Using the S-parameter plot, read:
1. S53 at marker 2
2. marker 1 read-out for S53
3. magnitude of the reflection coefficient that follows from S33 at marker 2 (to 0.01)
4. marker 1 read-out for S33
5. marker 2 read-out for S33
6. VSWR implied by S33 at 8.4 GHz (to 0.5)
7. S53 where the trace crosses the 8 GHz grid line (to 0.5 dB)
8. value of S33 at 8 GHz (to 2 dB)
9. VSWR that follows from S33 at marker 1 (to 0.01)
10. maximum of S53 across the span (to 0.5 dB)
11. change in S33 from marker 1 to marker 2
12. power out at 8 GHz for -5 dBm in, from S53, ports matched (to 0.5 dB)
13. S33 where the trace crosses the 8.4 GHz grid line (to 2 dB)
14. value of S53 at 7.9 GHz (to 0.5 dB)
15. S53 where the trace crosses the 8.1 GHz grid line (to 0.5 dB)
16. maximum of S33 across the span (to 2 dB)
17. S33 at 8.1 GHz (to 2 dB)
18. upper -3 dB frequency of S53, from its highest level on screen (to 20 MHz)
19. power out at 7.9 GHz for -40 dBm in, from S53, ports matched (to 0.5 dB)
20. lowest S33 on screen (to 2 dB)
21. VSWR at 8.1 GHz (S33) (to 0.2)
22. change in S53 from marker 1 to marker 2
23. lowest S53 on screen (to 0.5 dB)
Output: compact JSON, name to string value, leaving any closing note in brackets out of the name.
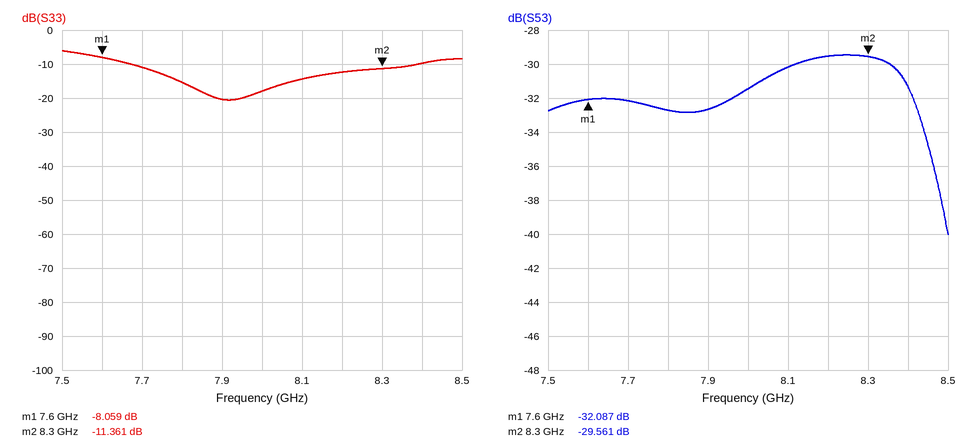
{"S53 at marker 2": "-29.561 dB", "marker 1 read-out for S53": "-32.087 dB", "magnitude of the reflection coefficient that follows from S33 at marker 2": "0.27", "marker 1 read-out for S33": "-8.059 dB", "marker 2 read-out for S33": "-11.361 dB", "VSWR implied by S33 at 8.4 GHz": "2.0", "S53 where the trace crosses the 8 GHz grid line": "-31.5 dB", "value of S33 at 8 GHz": "-18 dB", "VSWR that follows from S33 at marker 1": "2.31", "maximum of S53 across the span": "-29.5 dB", "change in S33 from marker 1 to marker 2": "-3.302 dB", "power out at 8 GHz for -5 dBm in, from S53, ports matched": "-36.5 dBm", "S33 where the trace crosses the 8.4 GHz grid line": "-10 dB", "value of S53 at 7.9 GHz": "-32.5 dB", "S53 where the trace crosses the 8.1 GHz grid line": "-30.0 dB", "maximum of S33 across the span": "-6 dB", "S33 at 8.1 GHz": "-14 dB", "upper -3 dB frequency of S53, from its highest level on screen": "8.42 GHz", "power out at 7.9 GHz for -40 dBm in, from S53, ports matched": "-72.5 dBm", "lowest S33 on screen": "-20 dB", "VSWR at 8.1 GHz (S33)": "1.4", "change in S53 from marker 1 to marker 2": "2.526 dB", "lowest S53 on screen": "-40.0 dB"}
